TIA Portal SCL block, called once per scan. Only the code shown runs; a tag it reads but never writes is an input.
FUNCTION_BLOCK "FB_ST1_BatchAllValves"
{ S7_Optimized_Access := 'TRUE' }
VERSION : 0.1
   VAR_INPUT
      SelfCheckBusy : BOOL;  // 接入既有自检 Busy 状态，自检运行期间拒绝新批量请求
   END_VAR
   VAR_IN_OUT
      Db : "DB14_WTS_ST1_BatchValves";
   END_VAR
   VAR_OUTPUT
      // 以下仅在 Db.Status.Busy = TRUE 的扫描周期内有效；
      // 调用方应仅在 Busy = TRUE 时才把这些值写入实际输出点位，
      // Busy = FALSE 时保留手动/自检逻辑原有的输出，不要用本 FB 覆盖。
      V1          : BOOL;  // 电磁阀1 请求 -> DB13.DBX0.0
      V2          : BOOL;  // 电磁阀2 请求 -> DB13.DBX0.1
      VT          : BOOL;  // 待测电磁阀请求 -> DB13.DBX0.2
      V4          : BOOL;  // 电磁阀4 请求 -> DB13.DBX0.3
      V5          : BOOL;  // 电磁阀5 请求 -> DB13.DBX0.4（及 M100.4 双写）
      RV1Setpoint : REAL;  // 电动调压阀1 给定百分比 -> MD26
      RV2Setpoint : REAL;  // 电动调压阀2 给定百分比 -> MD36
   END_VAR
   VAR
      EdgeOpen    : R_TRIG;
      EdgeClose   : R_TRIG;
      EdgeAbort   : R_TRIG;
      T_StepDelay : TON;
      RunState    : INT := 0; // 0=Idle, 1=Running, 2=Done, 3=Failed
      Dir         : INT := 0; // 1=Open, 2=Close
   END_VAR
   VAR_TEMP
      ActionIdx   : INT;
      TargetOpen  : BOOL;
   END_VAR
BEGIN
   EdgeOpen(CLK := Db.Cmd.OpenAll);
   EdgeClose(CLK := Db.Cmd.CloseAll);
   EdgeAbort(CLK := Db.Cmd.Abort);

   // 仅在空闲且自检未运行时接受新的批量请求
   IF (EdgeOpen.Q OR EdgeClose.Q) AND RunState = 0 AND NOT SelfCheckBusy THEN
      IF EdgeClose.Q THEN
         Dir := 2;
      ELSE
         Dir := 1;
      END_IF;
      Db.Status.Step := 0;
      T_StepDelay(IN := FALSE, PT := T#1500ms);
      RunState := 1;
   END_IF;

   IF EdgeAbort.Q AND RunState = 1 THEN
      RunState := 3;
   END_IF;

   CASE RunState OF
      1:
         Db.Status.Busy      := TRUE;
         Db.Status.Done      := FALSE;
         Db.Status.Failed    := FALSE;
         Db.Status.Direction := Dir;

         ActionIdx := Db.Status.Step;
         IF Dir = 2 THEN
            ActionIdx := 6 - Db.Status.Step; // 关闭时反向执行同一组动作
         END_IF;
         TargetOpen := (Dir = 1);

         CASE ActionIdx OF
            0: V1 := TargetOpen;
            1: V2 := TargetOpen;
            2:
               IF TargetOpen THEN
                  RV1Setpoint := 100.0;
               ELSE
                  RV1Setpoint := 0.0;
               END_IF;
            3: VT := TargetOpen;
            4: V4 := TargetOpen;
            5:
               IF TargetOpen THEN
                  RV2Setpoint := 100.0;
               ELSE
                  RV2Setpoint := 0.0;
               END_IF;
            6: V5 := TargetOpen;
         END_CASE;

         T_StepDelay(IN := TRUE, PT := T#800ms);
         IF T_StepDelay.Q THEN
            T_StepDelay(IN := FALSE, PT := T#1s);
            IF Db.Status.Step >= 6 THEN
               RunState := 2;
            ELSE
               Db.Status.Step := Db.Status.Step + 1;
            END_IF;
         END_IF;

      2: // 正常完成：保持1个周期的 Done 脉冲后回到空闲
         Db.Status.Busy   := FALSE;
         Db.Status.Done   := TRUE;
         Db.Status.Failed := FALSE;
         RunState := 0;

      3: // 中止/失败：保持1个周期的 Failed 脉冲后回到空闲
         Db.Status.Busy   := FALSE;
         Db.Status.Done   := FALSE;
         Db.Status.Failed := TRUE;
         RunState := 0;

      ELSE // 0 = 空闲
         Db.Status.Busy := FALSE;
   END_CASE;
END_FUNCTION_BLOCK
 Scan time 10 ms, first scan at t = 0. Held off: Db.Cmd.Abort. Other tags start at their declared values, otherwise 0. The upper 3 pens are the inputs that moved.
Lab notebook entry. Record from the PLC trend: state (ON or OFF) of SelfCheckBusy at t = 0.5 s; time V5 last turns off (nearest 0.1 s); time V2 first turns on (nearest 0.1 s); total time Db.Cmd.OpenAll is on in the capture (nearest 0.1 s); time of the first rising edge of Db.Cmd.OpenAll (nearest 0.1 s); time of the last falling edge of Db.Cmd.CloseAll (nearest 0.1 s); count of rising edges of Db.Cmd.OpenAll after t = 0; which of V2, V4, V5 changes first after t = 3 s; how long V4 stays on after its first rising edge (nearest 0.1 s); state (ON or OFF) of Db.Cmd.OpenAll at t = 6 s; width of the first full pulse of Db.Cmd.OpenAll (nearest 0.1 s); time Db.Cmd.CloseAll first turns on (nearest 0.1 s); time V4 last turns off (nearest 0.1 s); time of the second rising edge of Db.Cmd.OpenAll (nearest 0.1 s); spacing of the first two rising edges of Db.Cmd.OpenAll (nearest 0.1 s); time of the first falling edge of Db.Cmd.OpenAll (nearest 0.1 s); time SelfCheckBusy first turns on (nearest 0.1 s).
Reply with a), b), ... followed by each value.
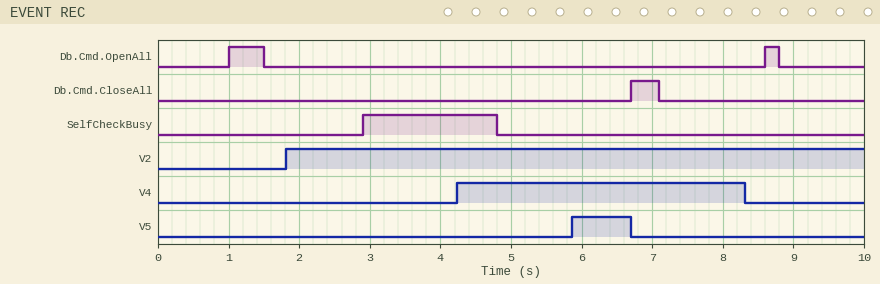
a) OFF
b) 6.7 s
c) 1.8 s
d) 0.7 s
e) 1.0 s
f) 7.1 s
g) 2
h) V4
i) 4.1 s
j) OFF
k) 0.5 s
l) 6.7 s
m) 8.3 s
n) 8.6 s
o) 7.6 s
p) 1.5 s
q) 2.9 s
